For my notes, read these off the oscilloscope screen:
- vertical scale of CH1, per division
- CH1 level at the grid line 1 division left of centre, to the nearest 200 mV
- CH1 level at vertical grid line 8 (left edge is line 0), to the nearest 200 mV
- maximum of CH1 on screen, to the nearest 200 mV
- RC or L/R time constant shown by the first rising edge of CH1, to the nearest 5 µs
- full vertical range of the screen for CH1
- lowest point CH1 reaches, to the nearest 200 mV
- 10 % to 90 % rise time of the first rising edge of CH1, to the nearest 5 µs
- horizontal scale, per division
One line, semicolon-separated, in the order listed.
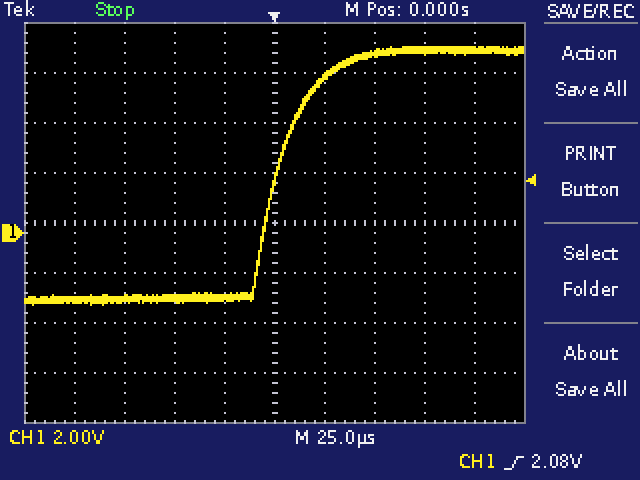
2 V; -2.6 V; 7.2 V; 7.4 V; 15 µs; 16 V; -2.8 V; 35 µs; 25 µs
